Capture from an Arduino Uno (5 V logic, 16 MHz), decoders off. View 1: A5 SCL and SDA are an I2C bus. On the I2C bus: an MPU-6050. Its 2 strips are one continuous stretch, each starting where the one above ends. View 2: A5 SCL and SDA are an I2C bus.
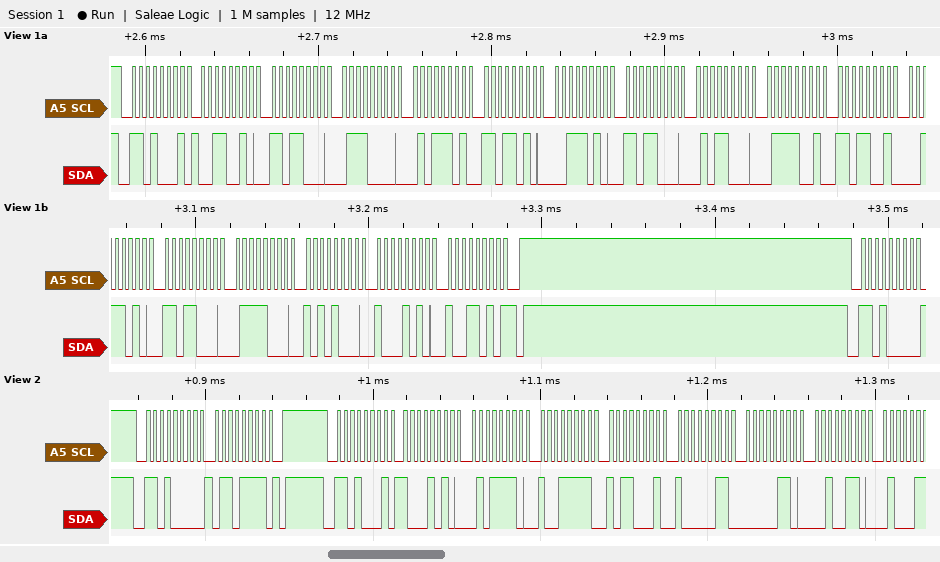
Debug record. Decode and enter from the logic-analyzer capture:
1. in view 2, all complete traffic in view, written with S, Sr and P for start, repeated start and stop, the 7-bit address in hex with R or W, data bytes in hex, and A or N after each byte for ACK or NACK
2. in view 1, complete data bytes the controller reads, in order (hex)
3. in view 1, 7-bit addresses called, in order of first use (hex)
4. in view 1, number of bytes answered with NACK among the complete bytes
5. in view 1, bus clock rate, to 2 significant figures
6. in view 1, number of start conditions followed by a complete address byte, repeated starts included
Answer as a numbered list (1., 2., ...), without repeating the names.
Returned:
1. S 68W A 6F A P S 68R A 8A A 5E A 9F A B1 A 83 A 06 A 26 A
2. 32 D8 70 5D DA 3A D8 58 79 D9 3A D8 78 A8 8A 9A
3. 0x68
4. 1
5. 250 kHz
6. 2
